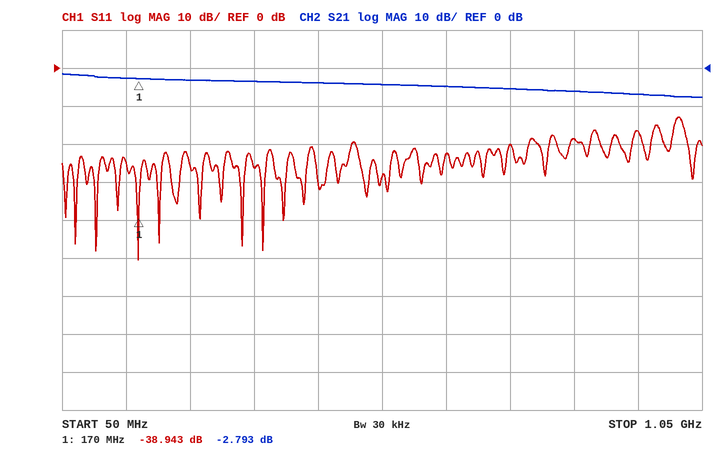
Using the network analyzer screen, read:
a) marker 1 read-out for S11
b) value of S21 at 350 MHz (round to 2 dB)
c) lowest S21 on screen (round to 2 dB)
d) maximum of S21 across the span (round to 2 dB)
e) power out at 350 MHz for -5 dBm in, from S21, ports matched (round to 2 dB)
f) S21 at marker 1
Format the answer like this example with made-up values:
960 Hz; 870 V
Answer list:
-38.943 dB; -4 dB; -8 dB; -2 dB; -8 dBm; -2.793 dB
